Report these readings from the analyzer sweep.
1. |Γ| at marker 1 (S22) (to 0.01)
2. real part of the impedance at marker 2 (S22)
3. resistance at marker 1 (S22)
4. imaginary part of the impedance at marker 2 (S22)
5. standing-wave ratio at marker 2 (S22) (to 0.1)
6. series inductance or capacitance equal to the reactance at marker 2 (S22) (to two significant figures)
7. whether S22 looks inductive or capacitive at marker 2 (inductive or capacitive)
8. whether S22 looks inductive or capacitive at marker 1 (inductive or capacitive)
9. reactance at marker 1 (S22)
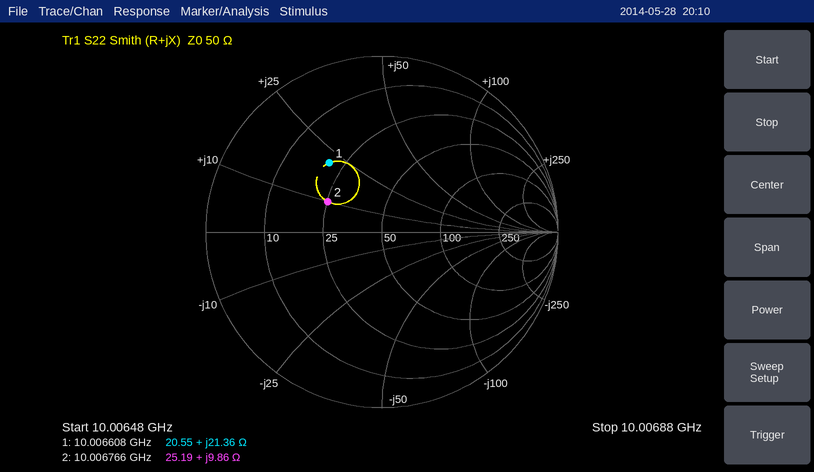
0.49
25.19 Ω
20.55 Ω
+9.86 Ω
2.1
160 pH
inductive
inductive
+21.36 Ω
